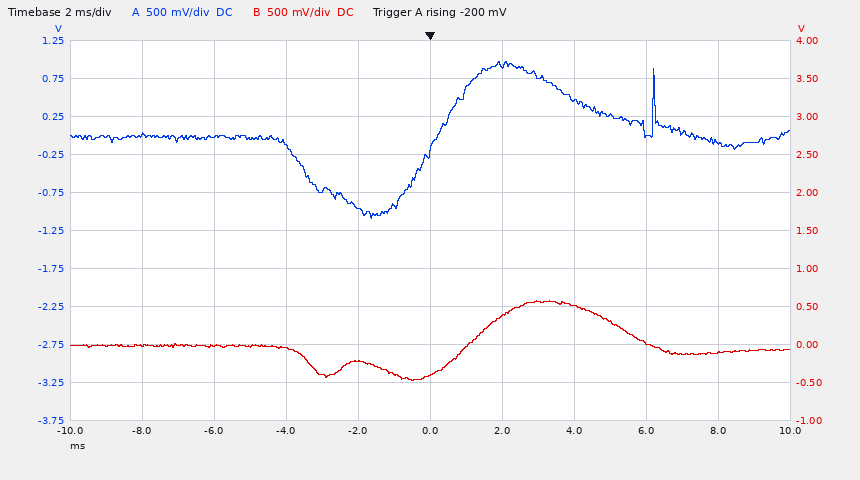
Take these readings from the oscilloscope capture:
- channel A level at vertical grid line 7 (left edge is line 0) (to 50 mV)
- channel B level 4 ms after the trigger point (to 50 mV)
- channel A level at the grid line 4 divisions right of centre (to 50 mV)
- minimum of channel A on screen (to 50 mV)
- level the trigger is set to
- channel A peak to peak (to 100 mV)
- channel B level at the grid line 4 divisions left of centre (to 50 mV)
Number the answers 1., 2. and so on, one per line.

1. 450 mV
2. 500 mV
3. -100 mV
4. -1.10 V
5. -200 mV
6. 2.10 V
7. 0 mV
